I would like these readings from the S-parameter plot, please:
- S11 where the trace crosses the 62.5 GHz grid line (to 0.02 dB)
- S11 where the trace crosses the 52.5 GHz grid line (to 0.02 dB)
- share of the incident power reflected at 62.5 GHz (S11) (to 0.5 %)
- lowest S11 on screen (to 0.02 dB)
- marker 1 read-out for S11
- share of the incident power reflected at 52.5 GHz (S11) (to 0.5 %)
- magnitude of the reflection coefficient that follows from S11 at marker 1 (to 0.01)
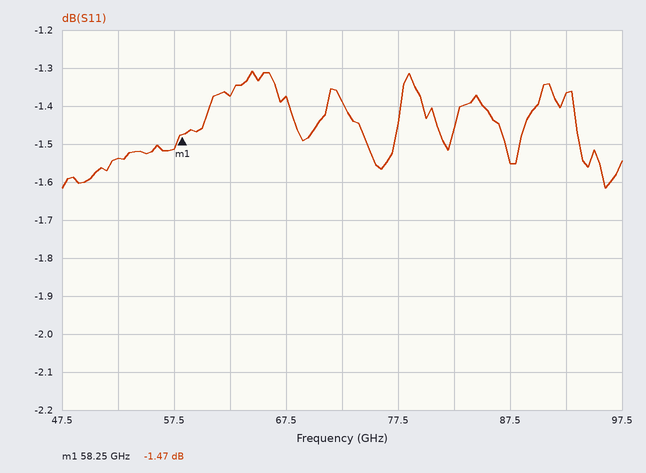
-1.38 dB
-1.54 dB
73.0 %
-1.62 dB
-1.47 dB
70.0 %
0.84
